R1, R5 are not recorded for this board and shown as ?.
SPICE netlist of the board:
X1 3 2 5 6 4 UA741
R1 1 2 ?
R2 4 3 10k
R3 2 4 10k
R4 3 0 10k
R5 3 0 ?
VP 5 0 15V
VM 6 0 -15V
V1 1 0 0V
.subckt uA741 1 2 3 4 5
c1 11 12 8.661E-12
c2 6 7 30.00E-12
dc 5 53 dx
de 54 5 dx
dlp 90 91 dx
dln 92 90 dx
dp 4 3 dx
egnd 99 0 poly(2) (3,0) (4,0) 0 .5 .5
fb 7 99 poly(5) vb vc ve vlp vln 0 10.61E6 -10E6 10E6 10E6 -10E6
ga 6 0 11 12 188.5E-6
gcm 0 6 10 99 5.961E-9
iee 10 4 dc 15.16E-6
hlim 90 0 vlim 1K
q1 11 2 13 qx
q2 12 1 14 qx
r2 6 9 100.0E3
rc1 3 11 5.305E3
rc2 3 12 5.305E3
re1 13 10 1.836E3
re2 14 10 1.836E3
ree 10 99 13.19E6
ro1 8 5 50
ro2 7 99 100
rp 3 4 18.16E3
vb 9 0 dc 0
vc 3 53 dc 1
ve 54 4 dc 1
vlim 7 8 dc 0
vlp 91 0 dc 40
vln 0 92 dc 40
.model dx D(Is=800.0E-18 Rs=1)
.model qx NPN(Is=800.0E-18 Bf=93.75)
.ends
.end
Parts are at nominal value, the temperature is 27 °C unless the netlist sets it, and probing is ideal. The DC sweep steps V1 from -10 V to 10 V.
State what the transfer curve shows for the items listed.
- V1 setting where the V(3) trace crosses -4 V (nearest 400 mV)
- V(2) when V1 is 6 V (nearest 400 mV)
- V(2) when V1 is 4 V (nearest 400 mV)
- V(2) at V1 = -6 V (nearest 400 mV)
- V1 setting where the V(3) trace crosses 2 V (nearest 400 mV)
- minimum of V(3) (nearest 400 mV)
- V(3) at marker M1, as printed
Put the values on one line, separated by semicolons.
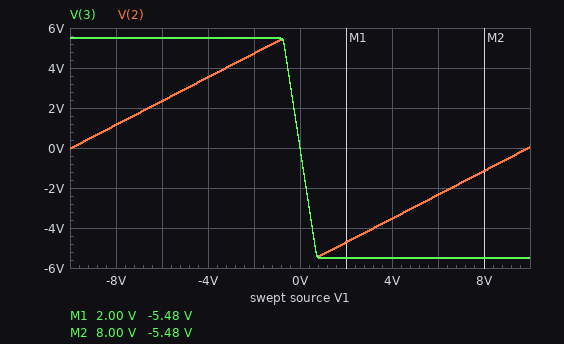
400 mV; -2.4 V; -3.6 V; 2.4 V; -400 mV; -5.6 V; -5.48 V
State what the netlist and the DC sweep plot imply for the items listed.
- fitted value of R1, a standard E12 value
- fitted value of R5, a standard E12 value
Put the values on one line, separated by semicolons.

6.8 kΩ; 15 kΩ
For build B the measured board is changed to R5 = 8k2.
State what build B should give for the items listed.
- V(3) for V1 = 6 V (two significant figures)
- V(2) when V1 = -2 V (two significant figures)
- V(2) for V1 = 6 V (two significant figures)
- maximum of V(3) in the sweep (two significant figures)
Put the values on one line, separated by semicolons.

-4.5 V; 3.9 V; -2.3 V; 4.5 V
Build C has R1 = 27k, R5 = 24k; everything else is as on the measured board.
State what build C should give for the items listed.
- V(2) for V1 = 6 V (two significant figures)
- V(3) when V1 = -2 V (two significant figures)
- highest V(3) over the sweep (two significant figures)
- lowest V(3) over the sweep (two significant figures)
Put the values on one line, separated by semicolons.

-2.1 V; 710 mV; 3.5 V; -3.5 V
